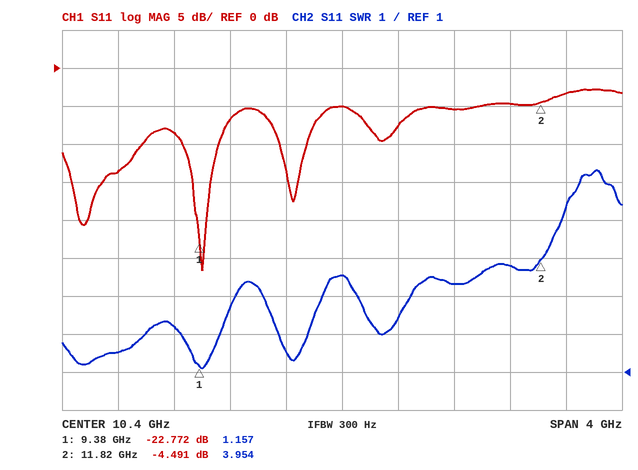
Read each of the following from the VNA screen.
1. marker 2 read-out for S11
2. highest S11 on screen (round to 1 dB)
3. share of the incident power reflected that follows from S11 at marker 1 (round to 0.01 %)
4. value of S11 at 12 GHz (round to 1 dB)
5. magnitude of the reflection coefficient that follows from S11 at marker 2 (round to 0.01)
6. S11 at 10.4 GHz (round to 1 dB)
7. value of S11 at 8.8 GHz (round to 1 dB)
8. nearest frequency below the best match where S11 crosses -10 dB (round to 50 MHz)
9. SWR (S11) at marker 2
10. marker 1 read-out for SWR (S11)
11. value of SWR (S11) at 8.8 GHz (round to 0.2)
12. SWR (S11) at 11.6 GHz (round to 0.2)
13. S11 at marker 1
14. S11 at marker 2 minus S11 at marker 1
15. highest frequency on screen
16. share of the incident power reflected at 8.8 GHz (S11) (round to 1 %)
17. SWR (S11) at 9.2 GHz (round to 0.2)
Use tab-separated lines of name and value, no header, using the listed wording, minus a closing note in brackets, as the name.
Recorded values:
marker 2 read-out for S11	-4.491 dB
highest S11 on screen	-3 dB
share of the incident power reflected that follows from S11 at marker 1	0.53 %
value of S11 at 12 GHz	-3 dB
magnitude of the reflection coefficient that follows from S11 at marker 2	0.60
S11 at 10.4 GHz	-5 dB
value of S11 at 8.8 GHz	-14 dB
nearest frequency below the best match where S11 crosses -10 dB	9.25 GHz
SWR (S11) at marker 2	3.954
marker 1 read-out for SWR	1.157
value of SWR (S11) at 8.8 GHz	1.6
SWR (S11) at 11.6 GHz	3.8
S11 at marker 1	-22.772 dB
S11 at marker 2 minus S11 at marker 1	18.281 dB
highest frequency on screen	12.4 GHz
share of the incident power reflected at 8.8 GHz (S11)	4 %
SWR (S11) at 9.2 GHz	2.2
